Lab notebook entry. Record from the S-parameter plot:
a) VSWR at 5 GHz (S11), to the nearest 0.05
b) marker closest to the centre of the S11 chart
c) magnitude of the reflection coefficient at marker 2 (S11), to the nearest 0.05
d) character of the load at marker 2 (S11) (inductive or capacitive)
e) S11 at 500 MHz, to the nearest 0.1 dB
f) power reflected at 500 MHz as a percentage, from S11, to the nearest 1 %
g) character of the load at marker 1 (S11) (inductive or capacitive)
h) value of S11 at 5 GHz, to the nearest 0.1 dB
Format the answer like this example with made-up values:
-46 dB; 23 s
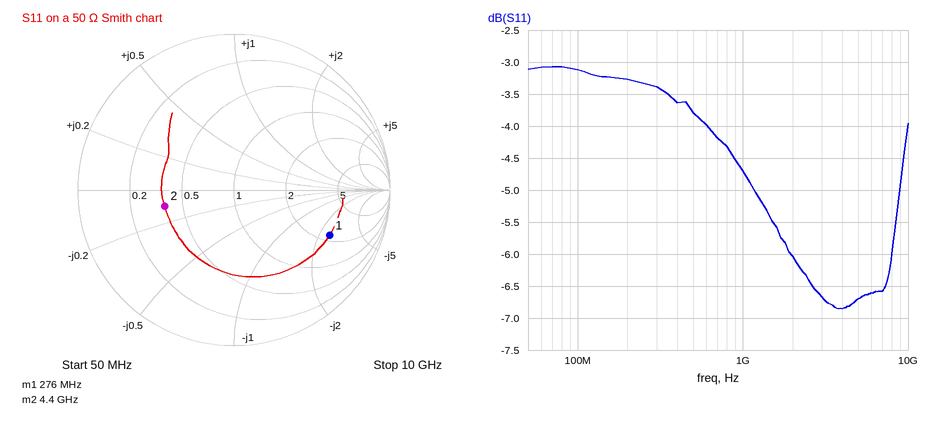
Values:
2.70; marker 2; 0.45; capacitive; -3.8 dB; 42 %; capacitive; -6.7 dB
